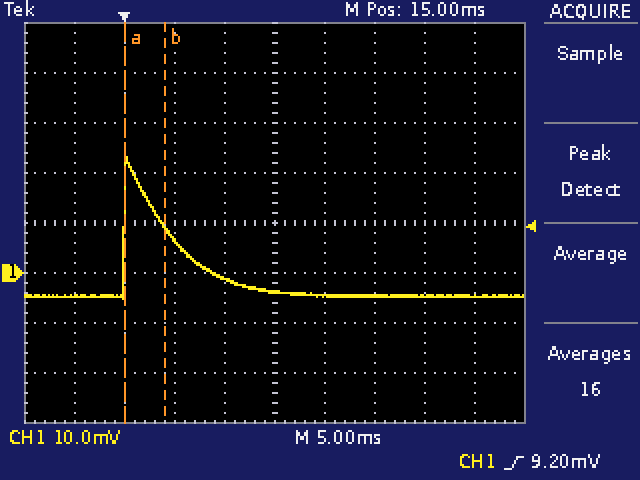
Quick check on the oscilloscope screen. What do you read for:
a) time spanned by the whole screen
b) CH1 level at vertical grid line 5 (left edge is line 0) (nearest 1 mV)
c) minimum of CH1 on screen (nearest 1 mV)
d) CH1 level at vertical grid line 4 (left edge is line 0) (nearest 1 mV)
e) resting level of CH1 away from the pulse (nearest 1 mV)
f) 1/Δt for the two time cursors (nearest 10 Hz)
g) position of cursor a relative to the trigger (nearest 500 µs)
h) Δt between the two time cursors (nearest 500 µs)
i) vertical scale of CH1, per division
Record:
50 ms
-4 mV
-5 mV
-1 mV
-5 mV
250 Hz
0.0 ms
4.0 ms
10 mV
